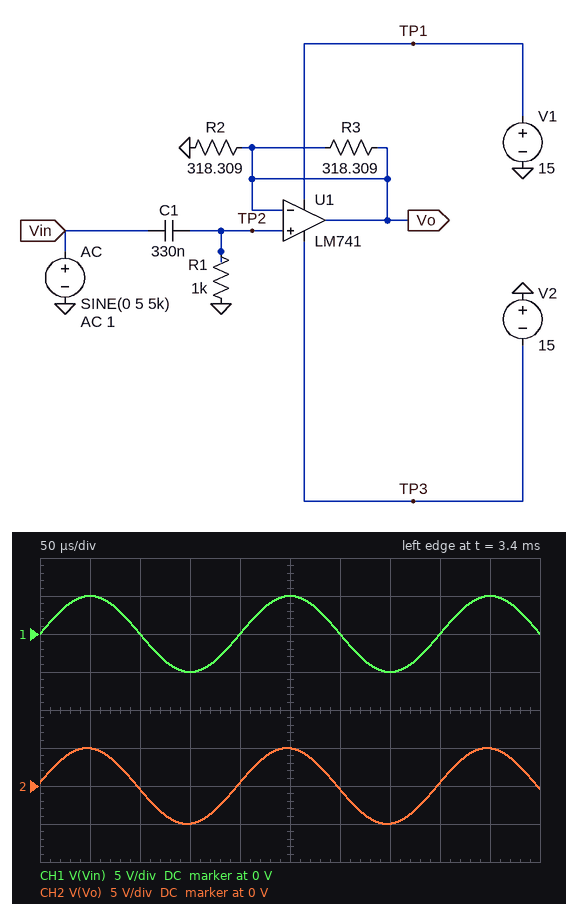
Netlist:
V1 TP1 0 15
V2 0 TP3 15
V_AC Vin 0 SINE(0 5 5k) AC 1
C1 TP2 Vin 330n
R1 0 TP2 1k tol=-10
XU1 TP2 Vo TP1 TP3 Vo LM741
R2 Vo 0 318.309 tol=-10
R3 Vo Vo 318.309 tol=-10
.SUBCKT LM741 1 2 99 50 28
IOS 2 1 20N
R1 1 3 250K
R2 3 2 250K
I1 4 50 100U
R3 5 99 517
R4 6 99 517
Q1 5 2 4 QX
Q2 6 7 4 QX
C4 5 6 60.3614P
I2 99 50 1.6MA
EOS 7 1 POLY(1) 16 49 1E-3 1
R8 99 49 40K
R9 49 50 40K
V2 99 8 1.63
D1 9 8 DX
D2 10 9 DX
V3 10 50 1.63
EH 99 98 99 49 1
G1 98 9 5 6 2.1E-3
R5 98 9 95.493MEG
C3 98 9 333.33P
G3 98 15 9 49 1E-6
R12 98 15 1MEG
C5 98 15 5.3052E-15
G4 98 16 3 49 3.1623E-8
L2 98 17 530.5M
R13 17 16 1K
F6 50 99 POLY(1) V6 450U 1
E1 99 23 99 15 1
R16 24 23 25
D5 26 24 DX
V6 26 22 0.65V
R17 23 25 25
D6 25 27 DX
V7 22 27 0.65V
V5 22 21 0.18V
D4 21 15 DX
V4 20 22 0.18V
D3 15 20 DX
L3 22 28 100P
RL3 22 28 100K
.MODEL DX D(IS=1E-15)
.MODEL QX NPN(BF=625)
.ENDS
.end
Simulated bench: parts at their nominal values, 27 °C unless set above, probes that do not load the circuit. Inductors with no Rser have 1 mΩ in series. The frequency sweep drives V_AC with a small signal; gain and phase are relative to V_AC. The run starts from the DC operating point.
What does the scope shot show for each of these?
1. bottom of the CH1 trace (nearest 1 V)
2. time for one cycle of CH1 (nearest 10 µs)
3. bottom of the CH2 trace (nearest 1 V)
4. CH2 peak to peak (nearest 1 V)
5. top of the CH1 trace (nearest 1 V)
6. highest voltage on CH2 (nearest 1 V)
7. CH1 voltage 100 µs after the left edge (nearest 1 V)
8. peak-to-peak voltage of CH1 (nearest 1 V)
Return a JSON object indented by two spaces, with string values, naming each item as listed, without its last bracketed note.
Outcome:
{
  "bottom of the CH1 trace": "-5 V",
  "time for one cycle of CH1": "200 µs",
  "bottom of the CH2 trace": "-5 V",
  "CH2 peak to peak": "10 V",
  "top of the CH1 trace": "5 V",
  "highest voltage on CH2": "5 V",
  "CH1 voltage 100 µs after the left edge": "0 V",
  "peak-to-peak voltage of CH1": "10 V"
}
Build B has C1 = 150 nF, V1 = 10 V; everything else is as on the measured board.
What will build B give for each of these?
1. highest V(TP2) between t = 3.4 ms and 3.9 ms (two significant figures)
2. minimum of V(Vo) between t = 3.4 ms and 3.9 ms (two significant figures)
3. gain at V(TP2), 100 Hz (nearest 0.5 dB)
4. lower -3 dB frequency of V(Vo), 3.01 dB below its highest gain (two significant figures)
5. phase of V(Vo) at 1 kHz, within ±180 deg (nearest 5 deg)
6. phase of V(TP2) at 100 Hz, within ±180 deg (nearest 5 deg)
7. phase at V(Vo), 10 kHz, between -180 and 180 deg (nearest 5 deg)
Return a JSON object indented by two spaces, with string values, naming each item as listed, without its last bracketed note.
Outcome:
{
  "highest V(TP2) between t = 3.4 ms and 3.9 ms": "4.9 V",
  "minimum of V(Vo) between t = 3.4 ms and 3.9 ms": "-4.9 V",
  "gain at V(TP2), 100 Hz": "-20.5 dB",
  "lower -3 dB frequency of V(Vo), 3.01 dB below its highest gain": "1.1 kHz",
  "phase of V(Vo) at 1 kHz, within ±180 deg": "45 deg",
  "phase of V(TP2) at 100 Hz, within ±180 deg": "85 deg",
  "phase at V(Vo), 10 kHz, between -180 and 180 deg": "5 deg"
}
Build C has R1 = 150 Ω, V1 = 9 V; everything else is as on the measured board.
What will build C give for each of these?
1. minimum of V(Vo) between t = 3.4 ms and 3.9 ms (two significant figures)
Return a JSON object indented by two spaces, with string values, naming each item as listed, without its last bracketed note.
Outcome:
{
  "minimum of V(Vo) between t = 3.4 ms and 3.9 ms": "-4.2 V"
}
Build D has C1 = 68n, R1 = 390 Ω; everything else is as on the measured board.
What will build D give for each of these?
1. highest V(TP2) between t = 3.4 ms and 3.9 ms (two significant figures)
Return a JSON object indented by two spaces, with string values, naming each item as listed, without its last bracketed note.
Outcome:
{
  "highest V(TP2) between t = 3.4 ms and 3.9 ms": "3.2 V"
}
